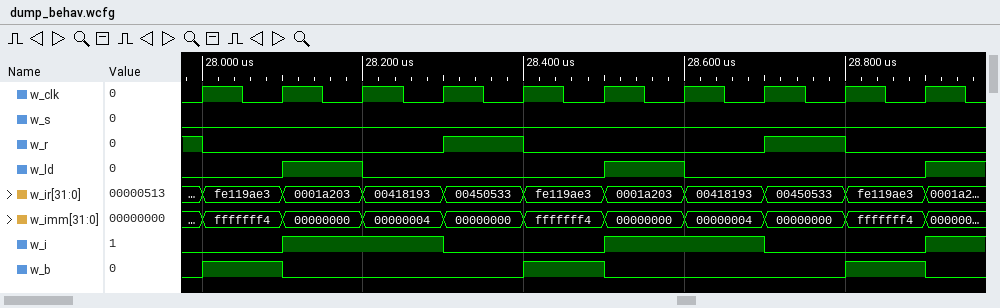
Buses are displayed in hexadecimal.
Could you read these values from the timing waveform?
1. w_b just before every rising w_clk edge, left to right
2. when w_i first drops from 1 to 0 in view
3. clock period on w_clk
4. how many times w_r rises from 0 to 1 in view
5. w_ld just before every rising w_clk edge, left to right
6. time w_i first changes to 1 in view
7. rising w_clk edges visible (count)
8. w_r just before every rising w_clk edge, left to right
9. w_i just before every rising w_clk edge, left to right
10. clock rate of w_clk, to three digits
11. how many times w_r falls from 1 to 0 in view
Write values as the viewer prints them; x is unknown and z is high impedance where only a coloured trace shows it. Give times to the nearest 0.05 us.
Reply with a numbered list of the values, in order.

1. 0 1 0 0 0 1 0 0 0 1
2. 28.3 us
3. 0.1 us
4. 2
5. 0 0 1 0 0 0 1 0 0 0
6. 28.1 us
7. 10
8. 1 0 0 0 1 0 0 0 1 0
9. 0 0 1 1 0 0 1 1 0 0
10. 10.0 MHz
11. 3
